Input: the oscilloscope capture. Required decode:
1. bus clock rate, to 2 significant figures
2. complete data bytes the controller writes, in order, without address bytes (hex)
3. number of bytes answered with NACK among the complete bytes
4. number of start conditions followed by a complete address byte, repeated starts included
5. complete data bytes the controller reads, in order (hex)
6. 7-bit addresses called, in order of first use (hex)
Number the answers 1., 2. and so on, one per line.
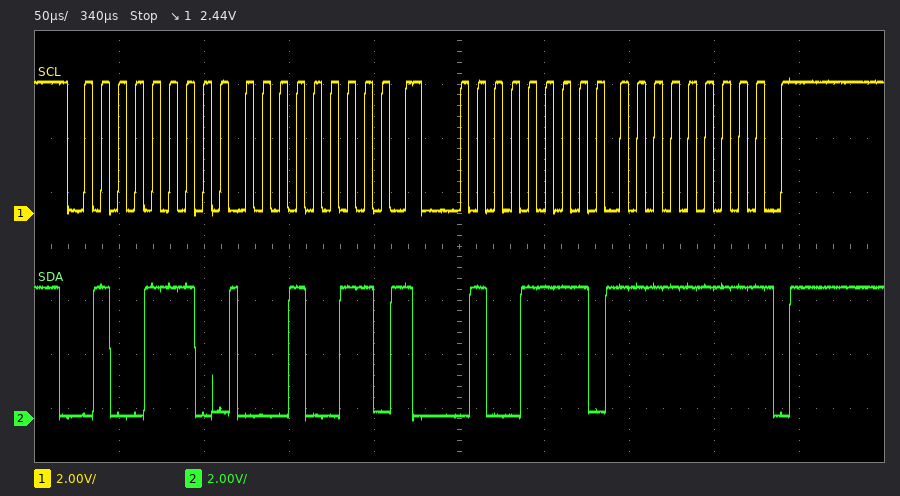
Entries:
1. 100 kHz
2. 13
3. 1
4. 2
5. FF
6. 0x27
